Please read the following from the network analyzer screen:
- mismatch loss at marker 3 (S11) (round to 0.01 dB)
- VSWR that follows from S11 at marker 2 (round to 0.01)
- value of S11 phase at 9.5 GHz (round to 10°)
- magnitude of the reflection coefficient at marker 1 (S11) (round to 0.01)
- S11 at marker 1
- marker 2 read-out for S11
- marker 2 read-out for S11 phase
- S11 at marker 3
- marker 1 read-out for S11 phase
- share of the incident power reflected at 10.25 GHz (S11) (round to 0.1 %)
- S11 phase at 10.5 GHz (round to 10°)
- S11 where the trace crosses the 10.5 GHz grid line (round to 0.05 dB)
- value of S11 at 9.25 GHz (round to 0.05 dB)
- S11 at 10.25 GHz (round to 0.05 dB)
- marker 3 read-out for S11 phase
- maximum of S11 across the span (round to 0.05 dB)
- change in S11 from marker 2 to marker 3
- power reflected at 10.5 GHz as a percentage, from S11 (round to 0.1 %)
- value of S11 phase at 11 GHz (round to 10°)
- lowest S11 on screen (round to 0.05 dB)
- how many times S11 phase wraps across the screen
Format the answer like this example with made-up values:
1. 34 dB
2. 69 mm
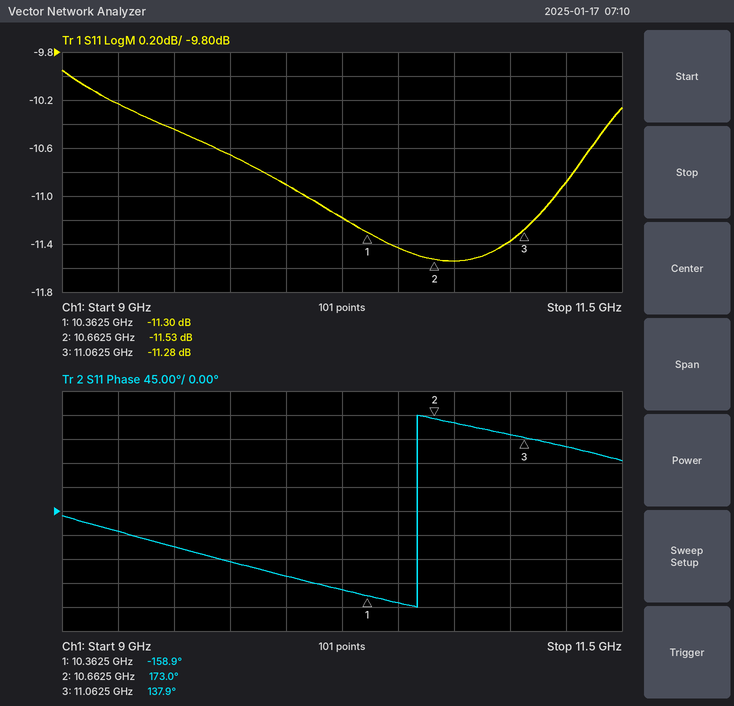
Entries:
1. 0.34 dB
2. 1.72
3. -70°
4. 0.27
5. -11.30 dB
6. -11.53 dB
7. 173.0°
8. -11.28 dB
9. -158.9°
10. 7.6 %
11. -170°
12. -11.45 dB
13. -10.25 dB
14. -11.20 dB
15. 137.9°
16. -9.95 dB
17. 0.25 dB
18. 7.2 %
19. 140°
20. -11.55 dB
21. 1
